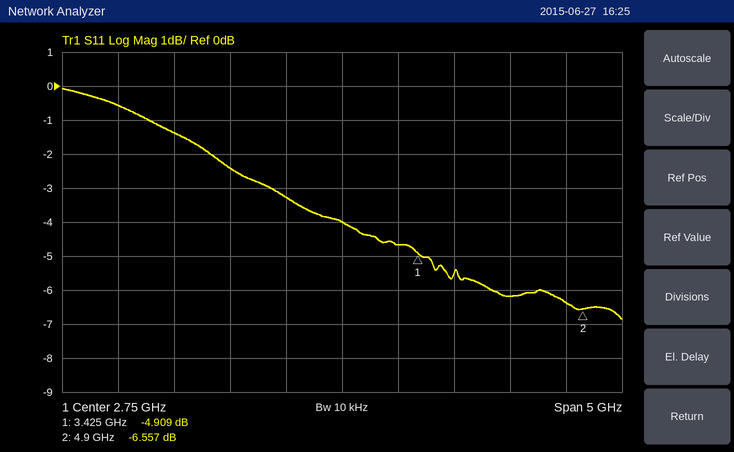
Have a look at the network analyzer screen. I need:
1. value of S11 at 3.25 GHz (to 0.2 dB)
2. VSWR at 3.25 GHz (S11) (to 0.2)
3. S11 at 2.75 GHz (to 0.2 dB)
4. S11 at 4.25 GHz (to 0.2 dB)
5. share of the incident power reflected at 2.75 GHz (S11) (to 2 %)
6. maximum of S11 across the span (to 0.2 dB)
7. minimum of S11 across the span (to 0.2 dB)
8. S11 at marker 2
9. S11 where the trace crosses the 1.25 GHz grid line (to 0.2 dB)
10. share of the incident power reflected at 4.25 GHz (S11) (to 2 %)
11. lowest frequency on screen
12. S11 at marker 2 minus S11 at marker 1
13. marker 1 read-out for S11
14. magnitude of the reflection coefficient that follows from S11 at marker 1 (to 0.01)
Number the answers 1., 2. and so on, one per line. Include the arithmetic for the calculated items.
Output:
1. -4.6 dB
2. |Γ| = 10^(-4.6/20) = 0.5888; VSWR = (1 + 0.5888)/(1 − 0.5888) ≈ 3.86, so 3.8 to the nearest 0.2
3. -4.0 dB
4. -6.2 dB
5. 10^(-4/10) ≈ 40 %
6. 0.0 dB
7. -6.8 dB
8. -6.557 dB
9. -1.4 dB
10. 10^(-6.2/10) ≈ 24 %
11. 250 MHz
12. -6.557 − (-4.909) = -1.648 dB
13. -4.909 dB
14. 10^(-4.909/20) ≈ 0.57
